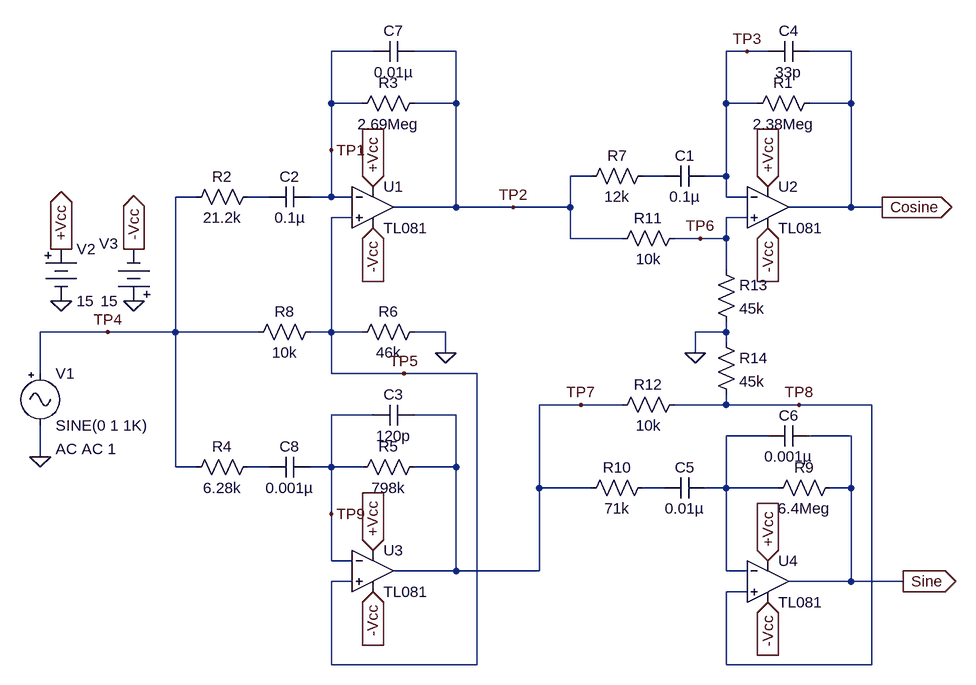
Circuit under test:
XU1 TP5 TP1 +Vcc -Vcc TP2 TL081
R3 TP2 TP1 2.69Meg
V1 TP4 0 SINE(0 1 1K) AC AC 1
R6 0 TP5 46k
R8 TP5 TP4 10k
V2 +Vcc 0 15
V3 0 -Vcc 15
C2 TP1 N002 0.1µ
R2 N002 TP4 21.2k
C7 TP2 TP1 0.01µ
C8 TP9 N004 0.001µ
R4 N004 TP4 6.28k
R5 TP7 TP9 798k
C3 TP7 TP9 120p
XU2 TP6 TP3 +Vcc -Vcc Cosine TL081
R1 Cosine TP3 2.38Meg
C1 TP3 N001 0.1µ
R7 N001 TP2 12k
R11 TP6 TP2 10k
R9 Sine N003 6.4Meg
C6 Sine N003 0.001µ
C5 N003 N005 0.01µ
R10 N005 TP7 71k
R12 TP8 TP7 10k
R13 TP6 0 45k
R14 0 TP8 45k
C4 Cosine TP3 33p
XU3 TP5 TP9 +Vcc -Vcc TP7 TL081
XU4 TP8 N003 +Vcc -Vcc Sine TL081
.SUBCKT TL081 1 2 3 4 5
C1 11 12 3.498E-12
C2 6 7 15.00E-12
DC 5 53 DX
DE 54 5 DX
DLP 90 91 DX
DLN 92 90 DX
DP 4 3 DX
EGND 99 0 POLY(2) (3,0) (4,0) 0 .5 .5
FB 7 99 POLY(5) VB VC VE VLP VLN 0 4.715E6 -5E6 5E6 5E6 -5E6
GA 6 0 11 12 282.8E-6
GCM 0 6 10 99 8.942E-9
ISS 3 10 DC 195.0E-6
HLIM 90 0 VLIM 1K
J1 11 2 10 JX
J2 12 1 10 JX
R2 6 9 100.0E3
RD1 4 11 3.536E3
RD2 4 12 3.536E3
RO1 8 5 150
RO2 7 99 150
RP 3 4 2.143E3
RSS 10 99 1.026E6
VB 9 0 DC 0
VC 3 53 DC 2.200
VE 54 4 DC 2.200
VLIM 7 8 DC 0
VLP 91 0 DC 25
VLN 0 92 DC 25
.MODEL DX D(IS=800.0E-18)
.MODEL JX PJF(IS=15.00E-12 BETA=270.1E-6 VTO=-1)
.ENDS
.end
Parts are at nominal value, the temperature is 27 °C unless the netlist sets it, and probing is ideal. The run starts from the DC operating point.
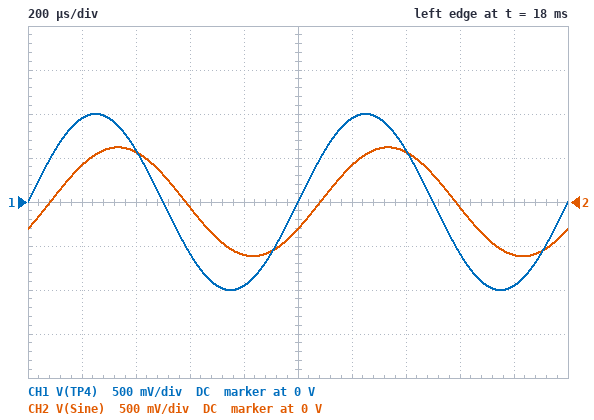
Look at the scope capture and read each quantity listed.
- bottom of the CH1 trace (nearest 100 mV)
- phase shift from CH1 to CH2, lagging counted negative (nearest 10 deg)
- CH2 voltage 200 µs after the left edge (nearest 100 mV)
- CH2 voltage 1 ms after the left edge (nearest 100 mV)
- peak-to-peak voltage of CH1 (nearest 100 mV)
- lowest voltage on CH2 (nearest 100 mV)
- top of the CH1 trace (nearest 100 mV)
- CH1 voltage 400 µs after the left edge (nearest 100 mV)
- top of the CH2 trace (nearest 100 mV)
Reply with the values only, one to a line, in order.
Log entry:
-1.0 V
-30 deg
400 mV
-300 mV
2.0 V
-600 mV
1.0 V
600 mV
600 mV
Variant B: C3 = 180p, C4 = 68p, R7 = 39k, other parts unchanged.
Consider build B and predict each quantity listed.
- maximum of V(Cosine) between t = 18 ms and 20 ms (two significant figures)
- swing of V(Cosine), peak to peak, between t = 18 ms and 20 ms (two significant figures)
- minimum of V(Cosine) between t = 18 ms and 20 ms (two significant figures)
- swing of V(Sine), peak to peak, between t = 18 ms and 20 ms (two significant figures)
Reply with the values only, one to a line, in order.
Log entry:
5.9 V
12 V
-5.9 V
970 mV
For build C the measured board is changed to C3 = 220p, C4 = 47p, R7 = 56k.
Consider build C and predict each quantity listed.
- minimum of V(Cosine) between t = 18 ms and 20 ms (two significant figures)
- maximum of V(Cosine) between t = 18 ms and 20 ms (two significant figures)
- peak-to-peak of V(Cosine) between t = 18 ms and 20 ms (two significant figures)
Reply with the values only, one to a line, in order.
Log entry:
-4.6 V
4.6 V
9.2 V
